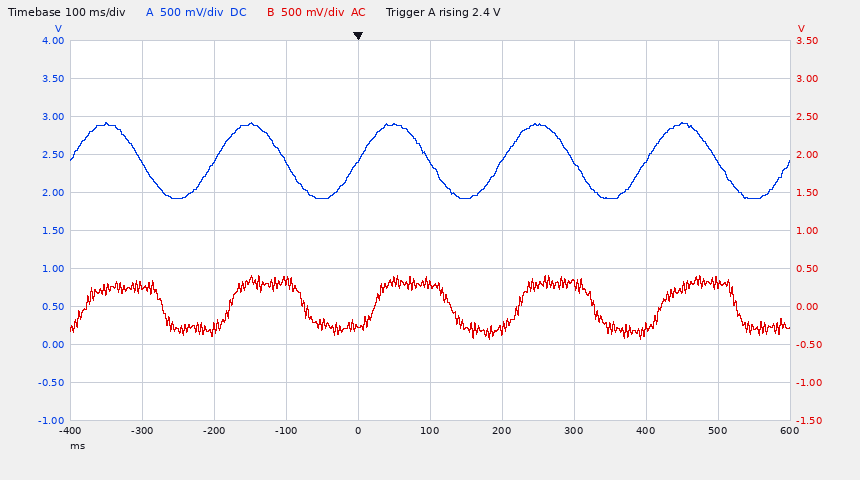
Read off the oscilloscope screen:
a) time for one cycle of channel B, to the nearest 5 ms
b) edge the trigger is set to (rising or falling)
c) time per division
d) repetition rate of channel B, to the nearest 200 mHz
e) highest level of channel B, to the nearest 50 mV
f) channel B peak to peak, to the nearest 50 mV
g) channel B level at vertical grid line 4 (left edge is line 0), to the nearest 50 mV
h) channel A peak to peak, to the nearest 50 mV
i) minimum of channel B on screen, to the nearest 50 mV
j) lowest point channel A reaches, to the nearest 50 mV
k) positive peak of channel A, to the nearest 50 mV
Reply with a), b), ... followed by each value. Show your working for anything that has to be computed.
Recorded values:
a) 200 ms
b) rising
c) 100 ms
d) 1 / 200 ms ≈ 5.0 Hz
e) 400 mV
f) 400 mV − (-450 mV) = 850 mV
g) -250 mV
h) 2.90 V − (1.90 V) = 1.00 V
i) -450 mV
j) 1.90 V
k) 2.90 V
